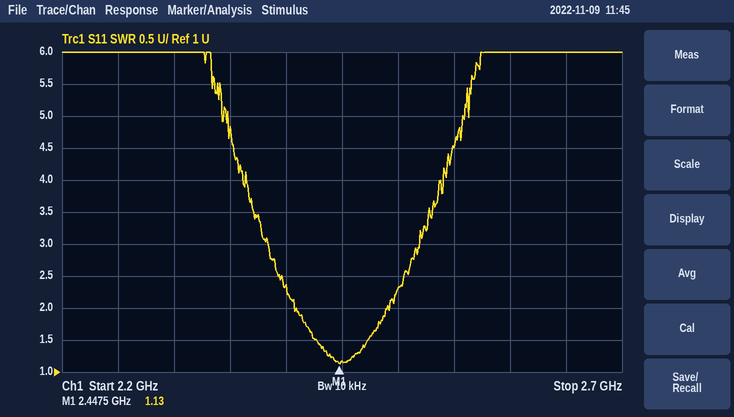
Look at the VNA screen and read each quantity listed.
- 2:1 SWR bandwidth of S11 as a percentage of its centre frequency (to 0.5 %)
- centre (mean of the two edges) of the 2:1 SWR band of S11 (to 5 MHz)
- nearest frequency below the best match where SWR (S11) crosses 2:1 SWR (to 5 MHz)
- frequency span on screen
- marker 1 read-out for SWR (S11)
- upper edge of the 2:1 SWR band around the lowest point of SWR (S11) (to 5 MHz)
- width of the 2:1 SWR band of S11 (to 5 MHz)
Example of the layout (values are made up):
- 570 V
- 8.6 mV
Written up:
- 3.5 %
- 2.450 GHz
- 2.410 GHz
- 500 MHz
- 1.13
- 2.490 GHz
- 80 MHz
